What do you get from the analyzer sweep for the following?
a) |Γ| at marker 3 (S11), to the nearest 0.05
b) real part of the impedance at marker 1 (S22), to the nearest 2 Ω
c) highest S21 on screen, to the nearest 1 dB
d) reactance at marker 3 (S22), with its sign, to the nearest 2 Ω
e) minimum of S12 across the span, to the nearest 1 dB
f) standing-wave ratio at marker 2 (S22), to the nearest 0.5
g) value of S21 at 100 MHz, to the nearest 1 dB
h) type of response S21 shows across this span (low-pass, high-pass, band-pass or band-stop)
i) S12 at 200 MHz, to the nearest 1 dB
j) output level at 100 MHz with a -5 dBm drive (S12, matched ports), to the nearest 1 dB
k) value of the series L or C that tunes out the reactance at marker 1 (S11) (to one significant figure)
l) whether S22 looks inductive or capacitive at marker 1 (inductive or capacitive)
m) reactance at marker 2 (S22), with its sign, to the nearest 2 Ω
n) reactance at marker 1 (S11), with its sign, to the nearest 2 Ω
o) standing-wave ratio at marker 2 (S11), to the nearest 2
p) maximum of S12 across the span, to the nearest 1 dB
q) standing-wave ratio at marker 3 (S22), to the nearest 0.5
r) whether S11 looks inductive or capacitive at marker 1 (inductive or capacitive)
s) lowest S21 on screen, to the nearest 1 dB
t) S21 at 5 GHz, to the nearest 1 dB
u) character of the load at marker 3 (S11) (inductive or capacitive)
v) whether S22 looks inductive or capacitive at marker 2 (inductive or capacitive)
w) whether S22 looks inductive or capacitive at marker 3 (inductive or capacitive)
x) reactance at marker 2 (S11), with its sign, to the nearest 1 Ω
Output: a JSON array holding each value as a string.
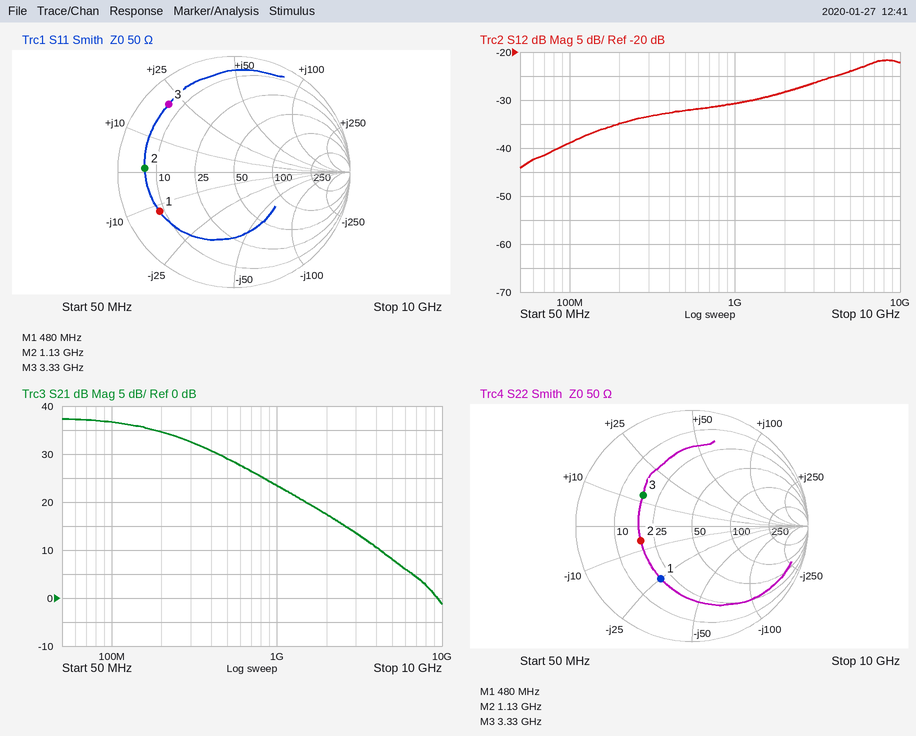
["0.80", "20 Ω", "37 dB", "+12 Ω", "-44 dB", "2.5", "37 dB", "low-pass", "-35 dB", "-44 dBm", "4 nH", "capacitive", "-6 Ω", "-12 Ω", "8", "-22 dB", "3.0", "capacitive", "-1 dB", "8 dB", "inductive", "capacitive", "inductive", "+1 Ω"]
